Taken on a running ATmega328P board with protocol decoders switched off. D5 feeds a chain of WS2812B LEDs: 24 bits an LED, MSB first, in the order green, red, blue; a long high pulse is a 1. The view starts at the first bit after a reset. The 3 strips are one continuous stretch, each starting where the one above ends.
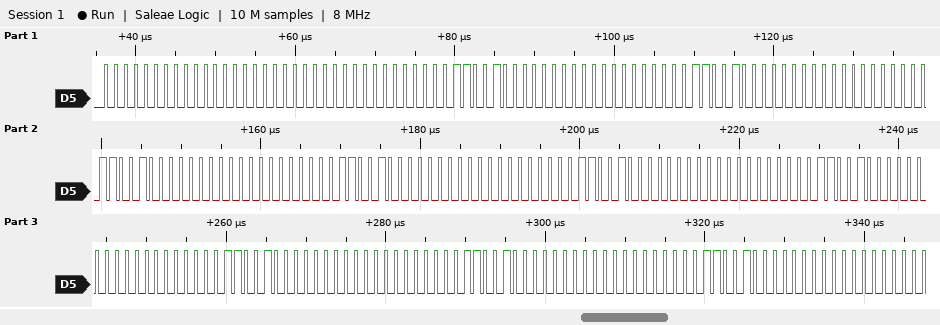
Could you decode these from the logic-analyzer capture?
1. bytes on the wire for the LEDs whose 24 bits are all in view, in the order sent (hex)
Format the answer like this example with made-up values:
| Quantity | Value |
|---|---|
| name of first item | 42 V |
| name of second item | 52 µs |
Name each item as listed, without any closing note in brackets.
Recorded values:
| Quantity | Value |
|---|---|
| bytes on the wire for the LEDs whose 24 bits are all in view, in the order sent | 00 00 00 00 19 00 00 19 00 00 19 00 00 19 00 00 19 00 00 19 00 00 19 00 00 19 00 00 19 00 |
